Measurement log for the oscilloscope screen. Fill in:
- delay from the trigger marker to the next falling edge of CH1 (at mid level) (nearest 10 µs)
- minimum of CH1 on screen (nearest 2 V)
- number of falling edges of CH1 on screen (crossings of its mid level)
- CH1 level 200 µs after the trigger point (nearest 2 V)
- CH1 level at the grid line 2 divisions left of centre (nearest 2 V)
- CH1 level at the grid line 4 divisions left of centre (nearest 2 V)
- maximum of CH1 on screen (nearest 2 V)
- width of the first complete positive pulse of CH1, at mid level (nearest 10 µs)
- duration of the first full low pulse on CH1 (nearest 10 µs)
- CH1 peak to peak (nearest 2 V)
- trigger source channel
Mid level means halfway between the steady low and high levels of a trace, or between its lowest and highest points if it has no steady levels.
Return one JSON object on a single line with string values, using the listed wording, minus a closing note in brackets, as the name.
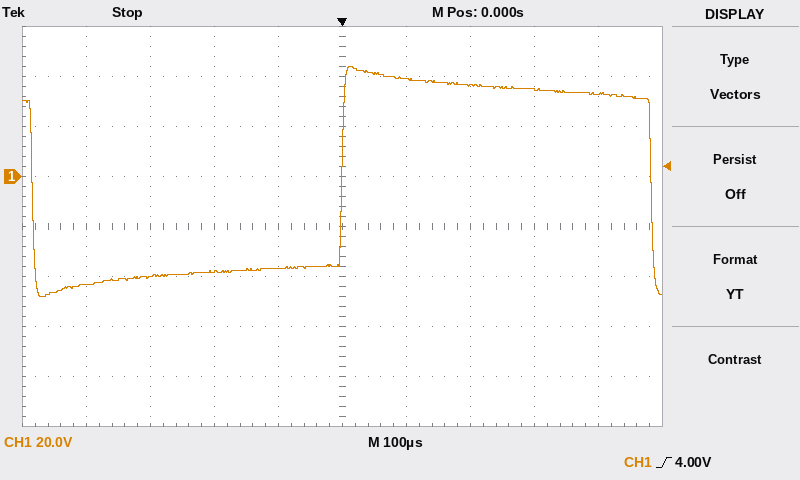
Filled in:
{"delay from the trigger marker to the next falling edge of CH1 (at mid level)": "480 µs", "minimum of CH1 on screen": "-48 V", "number of falling edges of CH1 on screen": "2", "CH1 level 200 µs after the trigger point": "36 V", "CH1 level at the grid line 2 divisions left of centre": "-38 V", "CH1 level at the grid line 4 divisions left of centre": "-44 V", "maximum of CH1 on screen": "44 V", "width of the first complete positive pulse of CH1, at mid level": "480 µs", "duration of the first full low pulse on CH1": "480 µs", "CH1 peak to peak": "92 V", "trigger source channel": "CH1"}
